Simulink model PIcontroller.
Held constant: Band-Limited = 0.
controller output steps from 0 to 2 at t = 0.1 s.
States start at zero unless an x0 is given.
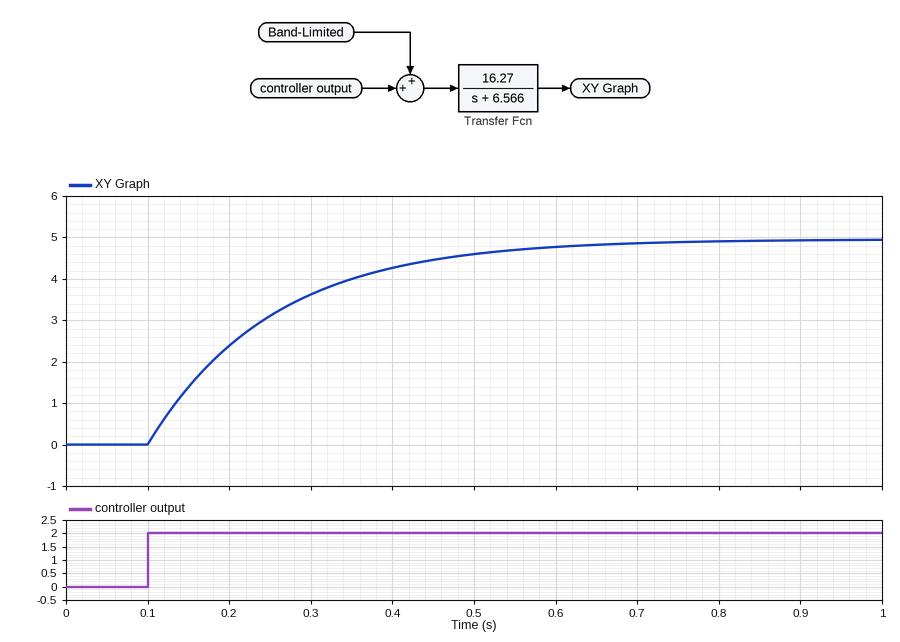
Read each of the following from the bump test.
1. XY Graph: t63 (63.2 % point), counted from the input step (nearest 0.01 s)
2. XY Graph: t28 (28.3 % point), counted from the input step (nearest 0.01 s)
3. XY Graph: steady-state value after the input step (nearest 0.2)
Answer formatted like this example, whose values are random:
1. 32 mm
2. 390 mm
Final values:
1. 0.15 s
2. 0.05 s
3. 5.0
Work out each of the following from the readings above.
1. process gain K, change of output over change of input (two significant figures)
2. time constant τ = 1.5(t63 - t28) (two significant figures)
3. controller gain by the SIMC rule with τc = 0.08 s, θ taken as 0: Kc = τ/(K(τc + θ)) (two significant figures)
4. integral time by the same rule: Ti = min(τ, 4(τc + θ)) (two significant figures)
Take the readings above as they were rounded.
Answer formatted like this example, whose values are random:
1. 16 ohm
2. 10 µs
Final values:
1. 2.5
2. 0.15 s
3. 0.75
4. 0.15 s
